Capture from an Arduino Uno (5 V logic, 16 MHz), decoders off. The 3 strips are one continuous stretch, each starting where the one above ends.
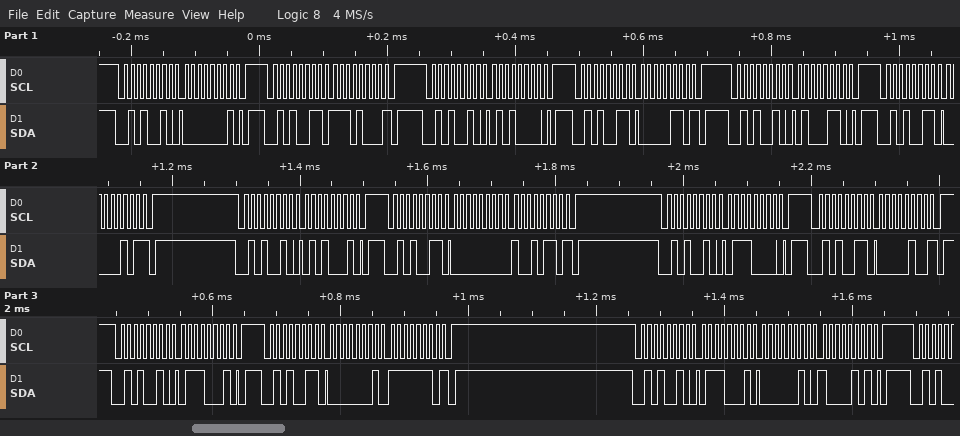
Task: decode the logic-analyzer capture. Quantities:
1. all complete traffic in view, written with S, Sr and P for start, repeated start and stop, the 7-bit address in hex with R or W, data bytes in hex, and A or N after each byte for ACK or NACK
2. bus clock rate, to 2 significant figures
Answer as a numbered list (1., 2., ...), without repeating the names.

1. S 29W A 01 A P S 29R A E8 N P S 29W A 50 A P S 29R A 06 N P S 29W A 46 A P S 29R A 05 N P S 29W A 51 A P S 29R A 00 A 96 N P S 29W A 70 A P S 29R A 04 N P S 29W A 71 A P S 29R A 01 A FE N P S 29W A 71 A 02 A 85 A P
2. 100 kHz
